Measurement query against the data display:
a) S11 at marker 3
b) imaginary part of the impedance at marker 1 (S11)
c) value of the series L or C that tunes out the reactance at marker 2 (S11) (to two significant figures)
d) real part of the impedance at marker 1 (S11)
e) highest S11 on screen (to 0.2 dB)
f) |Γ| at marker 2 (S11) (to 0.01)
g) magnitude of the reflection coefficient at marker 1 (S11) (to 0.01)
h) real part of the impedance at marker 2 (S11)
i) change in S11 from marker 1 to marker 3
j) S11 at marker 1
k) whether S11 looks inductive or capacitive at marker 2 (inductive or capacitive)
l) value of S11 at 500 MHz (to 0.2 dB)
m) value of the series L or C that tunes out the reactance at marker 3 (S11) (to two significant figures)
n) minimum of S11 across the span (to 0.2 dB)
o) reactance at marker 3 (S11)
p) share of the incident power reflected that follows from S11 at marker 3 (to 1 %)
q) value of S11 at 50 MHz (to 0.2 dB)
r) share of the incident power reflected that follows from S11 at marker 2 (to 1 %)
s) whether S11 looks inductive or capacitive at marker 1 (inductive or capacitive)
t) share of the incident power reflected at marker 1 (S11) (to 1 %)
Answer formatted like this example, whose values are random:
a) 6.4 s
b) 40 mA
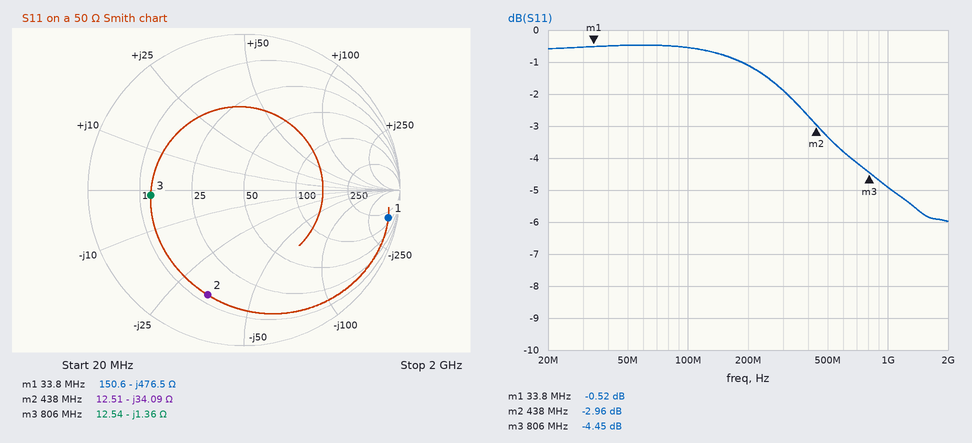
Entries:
a) -4.45 dB
b) -476.5 Ω
c) 12 nH
d) 150.6 Ω
e) -0.4 dB
f) 0.71
g) 0.94
h) 12.51 Ω
i) -3.93 dB
j) -0.52 dB
k) capacitive
l) -3.4 dB
m) 270 pH
n) -6.0 dB
o) -1.36 Ω
p) 36 %
q) -0.4 dB
r) 51 %
s) capacitive
t) 89 %
